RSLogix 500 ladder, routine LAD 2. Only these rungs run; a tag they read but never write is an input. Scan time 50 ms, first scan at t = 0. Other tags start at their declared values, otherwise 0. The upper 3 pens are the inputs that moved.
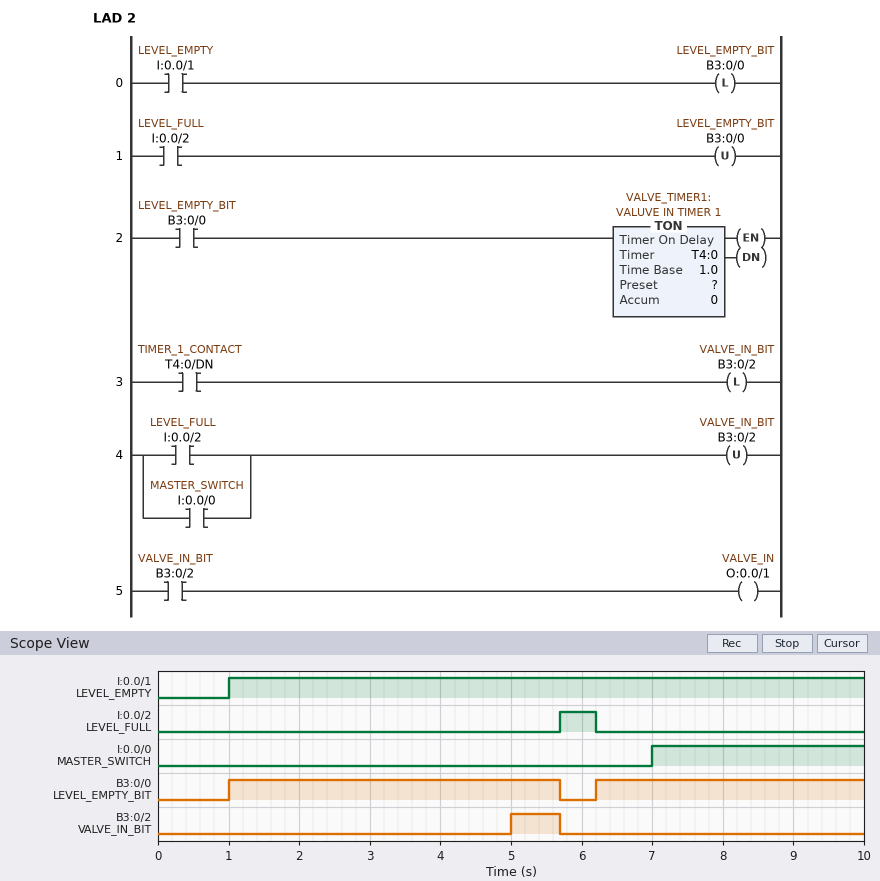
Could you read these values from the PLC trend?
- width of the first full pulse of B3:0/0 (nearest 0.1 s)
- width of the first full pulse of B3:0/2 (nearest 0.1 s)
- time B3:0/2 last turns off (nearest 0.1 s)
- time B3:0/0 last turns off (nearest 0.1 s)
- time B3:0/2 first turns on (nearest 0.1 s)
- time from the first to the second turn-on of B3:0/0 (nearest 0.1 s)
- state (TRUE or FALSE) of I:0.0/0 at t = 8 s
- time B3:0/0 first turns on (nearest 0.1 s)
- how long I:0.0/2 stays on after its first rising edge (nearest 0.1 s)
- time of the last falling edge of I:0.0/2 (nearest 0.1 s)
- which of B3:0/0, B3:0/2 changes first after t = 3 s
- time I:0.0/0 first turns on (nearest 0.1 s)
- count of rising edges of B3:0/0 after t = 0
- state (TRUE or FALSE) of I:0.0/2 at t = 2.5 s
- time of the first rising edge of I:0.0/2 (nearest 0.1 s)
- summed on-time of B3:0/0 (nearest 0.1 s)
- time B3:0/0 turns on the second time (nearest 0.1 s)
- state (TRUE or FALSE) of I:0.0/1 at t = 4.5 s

4.7 s
0.7 s
5.7 s
5.7 s
5.0 s
5.2 s
TRUE
1.0 s
0.5 s
6.2 s
B3:0/2
7.0 s
2
FALSE
5.7 s
8.5 s
6.2 s
TRUE
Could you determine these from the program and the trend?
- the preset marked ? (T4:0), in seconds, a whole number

4 s
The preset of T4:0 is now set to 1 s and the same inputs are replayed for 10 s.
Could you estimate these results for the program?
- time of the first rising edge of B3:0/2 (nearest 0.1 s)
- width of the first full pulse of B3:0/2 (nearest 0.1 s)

2.0 s
3.7 s
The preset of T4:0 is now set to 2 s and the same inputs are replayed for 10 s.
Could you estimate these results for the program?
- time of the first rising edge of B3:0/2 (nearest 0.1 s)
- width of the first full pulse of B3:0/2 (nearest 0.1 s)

3.0 s
2.7 s
